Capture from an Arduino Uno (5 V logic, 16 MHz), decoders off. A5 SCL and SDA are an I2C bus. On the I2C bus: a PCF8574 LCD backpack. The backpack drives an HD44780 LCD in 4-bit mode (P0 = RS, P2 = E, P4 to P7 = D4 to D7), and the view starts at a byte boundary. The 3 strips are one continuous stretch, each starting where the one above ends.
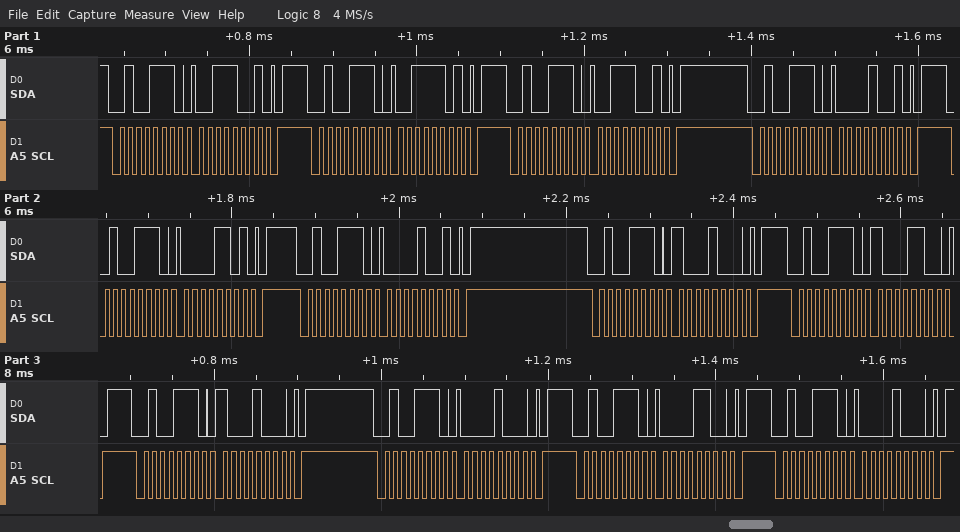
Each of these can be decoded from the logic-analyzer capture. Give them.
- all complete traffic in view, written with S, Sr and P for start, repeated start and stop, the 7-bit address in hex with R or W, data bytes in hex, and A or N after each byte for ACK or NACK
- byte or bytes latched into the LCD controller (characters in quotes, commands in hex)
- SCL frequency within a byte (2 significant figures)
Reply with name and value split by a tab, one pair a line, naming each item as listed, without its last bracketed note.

all complete traffic in view, written with S, Sr and P for start, repeated start and stop, the 7-bit address in hex with R or W, data bytes in hex, and A or N after each byte for ACK or NACK	S 27W A 39 A P S 27W A 3D A P S 27W A 39 A P S 27W A 09 A P S 27W A 0D A P S 27W A 09 A P S 27W A 88 A P S 27W A 8C A P S 27W A 88 A P S 27W A 08 A P S 27W A 0C A P S 27W A 08 A P
byte or bytes latched into the LCD controller	'0' 0x80
SCL frequency within a byte	100 kHz
